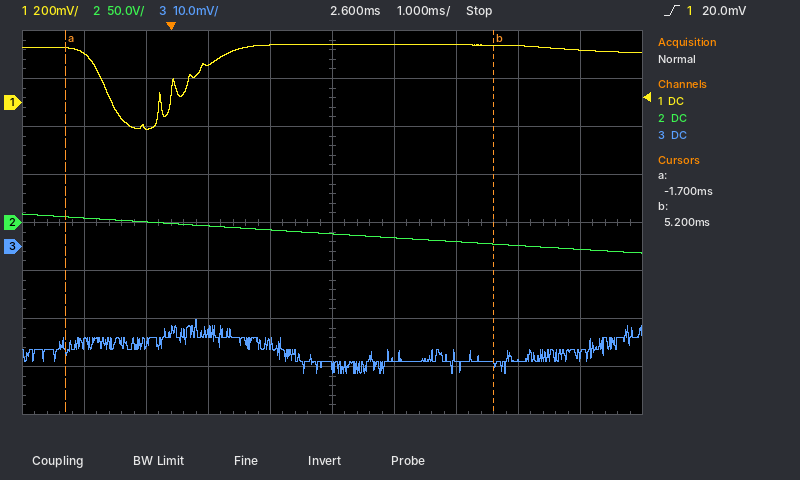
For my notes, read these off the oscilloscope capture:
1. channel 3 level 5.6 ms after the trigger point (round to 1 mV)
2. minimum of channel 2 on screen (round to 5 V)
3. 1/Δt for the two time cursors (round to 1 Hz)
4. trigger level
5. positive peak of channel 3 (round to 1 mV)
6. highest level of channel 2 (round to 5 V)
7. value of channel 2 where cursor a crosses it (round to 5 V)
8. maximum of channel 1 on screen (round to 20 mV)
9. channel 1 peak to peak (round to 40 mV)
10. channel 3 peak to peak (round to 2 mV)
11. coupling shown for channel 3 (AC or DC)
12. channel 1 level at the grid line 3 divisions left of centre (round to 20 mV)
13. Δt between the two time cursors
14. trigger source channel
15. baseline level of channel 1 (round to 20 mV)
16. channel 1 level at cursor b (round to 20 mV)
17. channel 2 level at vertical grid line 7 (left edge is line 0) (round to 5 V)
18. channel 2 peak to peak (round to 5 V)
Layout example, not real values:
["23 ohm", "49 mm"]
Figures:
["-24 mV", "-30 V", "145 Hz", "20.0 mV", "-15 mV", "10 V", "5 V", "240 mV", "360 mV", "12 mV", "DC", "-100 mV", "6.9 ms", "channel 1", "240 mV", "240 mV", "-20 V", "40 V"]
